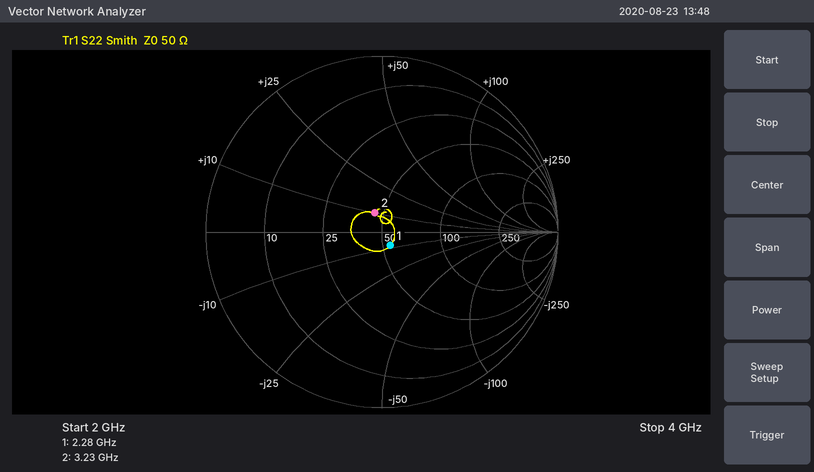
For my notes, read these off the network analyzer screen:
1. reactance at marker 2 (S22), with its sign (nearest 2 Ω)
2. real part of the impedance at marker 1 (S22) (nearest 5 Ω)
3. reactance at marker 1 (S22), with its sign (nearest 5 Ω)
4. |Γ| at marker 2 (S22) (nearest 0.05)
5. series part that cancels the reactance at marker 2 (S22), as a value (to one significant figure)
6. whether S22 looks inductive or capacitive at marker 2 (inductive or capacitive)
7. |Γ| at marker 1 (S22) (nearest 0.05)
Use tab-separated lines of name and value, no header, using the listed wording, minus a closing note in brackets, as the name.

reactance at marker 2 (S22), with its sign	+10 Ω
real part of the impedance at marker 1 (S22)	55 Ω
reactance at marker 1 (S22), with its sign	-10 Ω
|Γ| at marker 2 (S22)	0.10
series part that cancels the reactance at marker 2 (S22), as a value	5 pF
whether S22 looks inductive or capacitive at marker 2	inductive
|Γ| at marker 1 (S22)	0.10
